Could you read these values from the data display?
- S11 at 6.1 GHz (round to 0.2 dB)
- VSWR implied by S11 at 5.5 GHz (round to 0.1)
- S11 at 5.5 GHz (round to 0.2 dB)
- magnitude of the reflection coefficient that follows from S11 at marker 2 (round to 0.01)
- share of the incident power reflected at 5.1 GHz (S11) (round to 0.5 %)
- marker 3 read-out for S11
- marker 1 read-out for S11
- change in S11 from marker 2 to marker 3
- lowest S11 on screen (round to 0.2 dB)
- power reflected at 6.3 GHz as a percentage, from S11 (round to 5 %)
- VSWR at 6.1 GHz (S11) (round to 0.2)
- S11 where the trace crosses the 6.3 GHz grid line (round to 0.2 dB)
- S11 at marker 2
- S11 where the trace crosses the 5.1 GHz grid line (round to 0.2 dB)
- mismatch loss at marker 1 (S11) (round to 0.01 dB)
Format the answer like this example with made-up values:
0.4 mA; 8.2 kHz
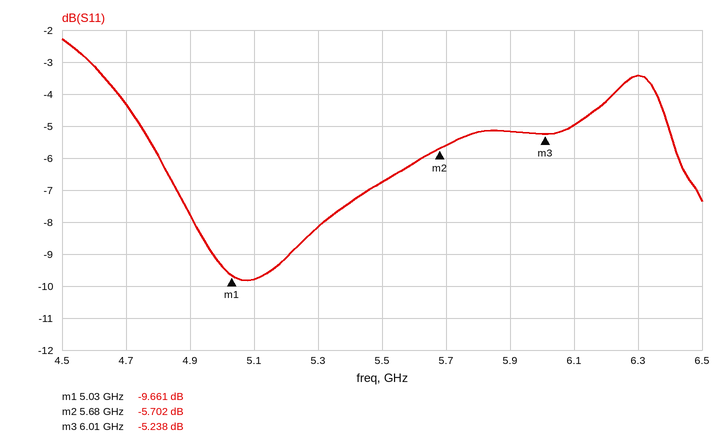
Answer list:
-5.0 dB; 2.7; -6.8 dB; 0.52; 10.5 %; -5.238 dB; -9.661 dB; 0.464 dB; -9.8 dB; 45 %; 3.6; -3.4 dB; -5.702 dB; -9.8 dB; 0.50 dB
